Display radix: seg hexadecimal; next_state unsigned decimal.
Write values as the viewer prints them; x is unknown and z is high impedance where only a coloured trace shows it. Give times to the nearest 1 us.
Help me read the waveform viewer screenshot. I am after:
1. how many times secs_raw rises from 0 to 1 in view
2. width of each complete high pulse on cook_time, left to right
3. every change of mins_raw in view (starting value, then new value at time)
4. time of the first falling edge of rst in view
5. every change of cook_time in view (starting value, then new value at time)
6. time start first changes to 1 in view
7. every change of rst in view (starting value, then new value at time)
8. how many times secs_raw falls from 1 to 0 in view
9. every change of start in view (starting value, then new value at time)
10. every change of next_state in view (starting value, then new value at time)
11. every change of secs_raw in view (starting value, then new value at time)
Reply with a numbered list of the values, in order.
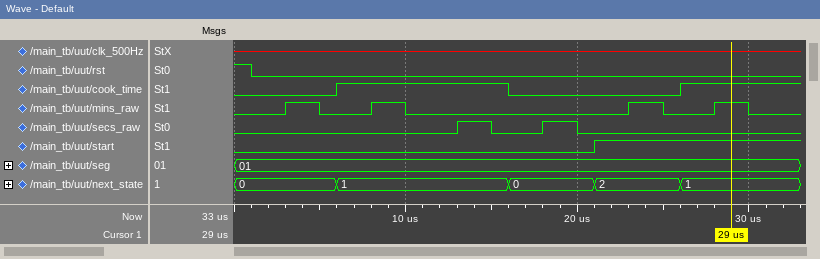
1. 2
2. 10 us
3. 0, 1 at 3 us, 0 at 5 us, 1 at 8 us, 0 at 10 us, 1 at 23 us, 0 at 25 us, 1 at 28 us, 0 at 30 us
4. 1 us
5. 0, 1 at 6 us, 0 at 16 us, 1 at 26 us
6. 21 us
7. 1, 0 at 1 us
8. 2
9. 0, 1 at 21 us
10. 0, 1 at 6 us, 0 at 16 us, 2 at 21 us, 1 at 26 us
11. 0, 1 at 13 us, 0 at 15 us, 1 at 18 us, 0 at 20 us
